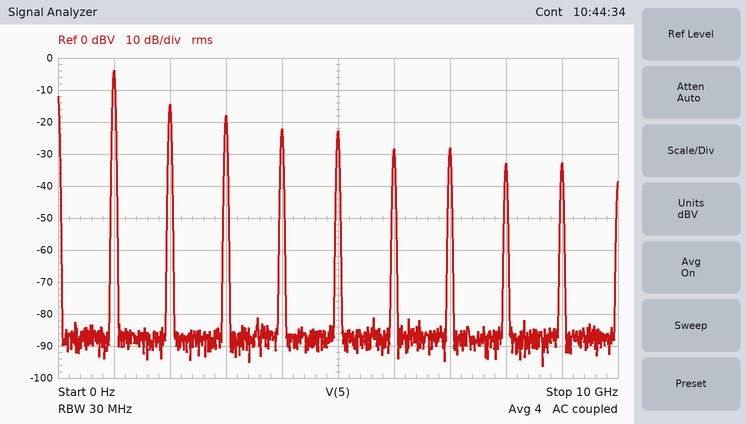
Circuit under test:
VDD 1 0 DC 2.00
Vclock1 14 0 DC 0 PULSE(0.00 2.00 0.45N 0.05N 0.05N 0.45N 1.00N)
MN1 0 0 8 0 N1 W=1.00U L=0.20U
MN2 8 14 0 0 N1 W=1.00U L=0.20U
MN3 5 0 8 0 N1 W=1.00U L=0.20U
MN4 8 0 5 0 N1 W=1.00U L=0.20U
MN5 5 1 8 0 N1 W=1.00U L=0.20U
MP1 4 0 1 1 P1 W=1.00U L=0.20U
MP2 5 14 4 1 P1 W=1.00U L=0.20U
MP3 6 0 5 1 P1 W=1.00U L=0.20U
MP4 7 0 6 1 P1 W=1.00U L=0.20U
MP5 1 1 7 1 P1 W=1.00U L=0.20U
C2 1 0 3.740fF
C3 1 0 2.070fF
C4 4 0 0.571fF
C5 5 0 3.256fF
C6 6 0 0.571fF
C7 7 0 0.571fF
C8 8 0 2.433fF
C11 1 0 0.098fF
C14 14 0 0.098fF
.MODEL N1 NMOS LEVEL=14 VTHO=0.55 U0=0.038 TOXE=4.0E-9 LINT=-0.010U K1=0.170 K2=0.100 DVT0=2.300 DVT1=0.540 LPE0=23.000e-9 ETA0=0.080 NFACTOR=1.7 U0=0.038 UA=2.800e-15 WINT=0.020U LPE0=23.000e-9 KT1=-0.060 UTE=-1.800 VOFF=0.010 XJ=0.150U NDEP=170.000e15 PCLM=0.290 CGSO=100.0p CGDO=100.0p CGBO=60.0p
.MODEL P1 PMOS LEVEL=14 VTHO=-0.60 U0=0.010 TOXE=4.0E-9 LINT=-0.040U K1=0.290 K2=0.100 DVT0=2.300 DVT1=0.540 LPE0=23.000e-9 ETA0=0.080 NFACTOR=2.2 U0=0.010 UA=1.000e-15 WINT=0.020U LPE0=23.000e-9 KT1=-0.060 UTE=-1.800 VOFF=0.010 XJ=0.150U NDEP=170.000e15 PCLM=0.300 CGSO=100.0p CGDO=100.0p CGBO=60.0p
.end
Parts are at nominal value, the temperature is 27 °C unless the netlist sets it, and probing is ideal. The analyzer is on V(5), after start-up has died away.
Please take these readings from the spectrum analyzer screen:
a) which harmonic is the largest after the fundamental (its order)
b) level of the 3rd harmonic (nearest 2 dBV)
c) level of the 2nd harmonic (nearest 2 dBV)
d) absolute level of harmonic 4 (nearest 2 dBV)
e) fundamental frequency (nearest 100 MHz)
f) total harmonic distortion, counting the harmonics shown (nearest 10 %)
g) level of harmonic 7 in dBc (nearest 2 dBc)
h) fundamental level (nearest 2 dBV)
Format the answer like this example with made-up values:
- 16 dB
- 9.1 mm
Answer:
- 2
- -18 dBV
- -14 dBV
- -22 dBV
- 1.0 GHz
- 40 %
- -24 dBc
- -4 dBV
